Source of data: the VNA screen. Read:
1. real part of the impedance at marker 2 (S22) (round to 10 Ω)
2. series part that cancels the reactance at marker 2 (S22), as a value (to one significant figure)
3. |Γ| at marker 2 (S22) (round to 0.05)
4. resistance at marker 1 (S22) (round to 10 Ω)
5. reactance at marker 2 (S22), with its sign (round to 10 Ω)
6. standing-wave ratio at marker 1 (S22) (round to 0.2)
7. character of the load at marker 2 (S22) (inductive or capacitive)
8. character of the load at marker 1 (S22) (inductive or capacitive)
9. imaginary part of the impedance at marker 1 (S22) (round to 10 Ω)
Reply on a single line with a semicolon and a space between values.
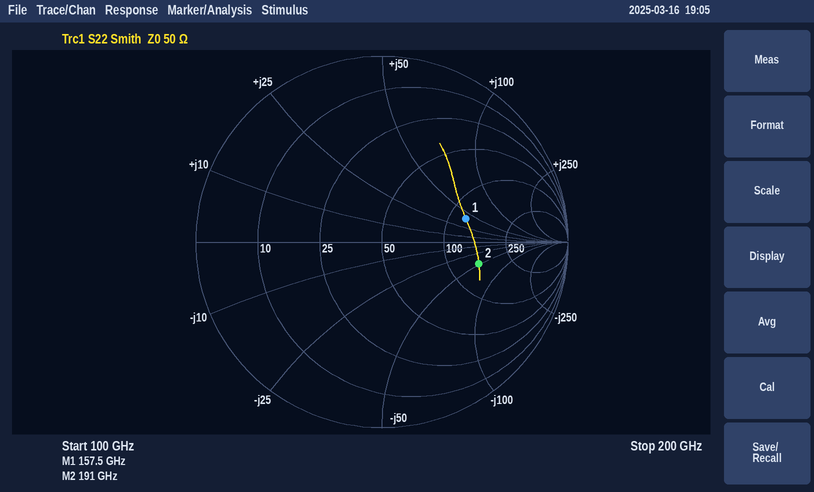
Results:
150 Ω; 40 pH; 0.55; 120 Ω; -50 Ω; 2.8; capacitive; inductive; +40 Ω
